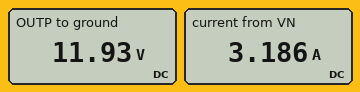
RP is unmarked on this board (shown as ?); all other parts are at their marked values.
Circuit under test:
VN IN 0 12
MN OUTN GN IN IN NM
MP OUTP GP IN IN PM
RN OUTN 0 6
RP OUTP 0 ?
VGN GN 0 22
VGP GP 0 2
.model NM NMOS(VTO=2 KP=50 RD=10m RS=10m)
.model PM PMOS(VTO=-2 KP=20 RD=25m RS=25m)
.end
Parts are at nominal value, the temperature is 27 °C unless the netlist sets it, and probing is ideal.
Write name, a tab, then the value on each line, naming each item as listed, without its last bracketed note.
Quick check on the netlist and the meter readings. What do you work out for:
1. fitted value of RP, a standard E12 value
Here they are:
fitted value of RP, a standard E12 value	10 Ω
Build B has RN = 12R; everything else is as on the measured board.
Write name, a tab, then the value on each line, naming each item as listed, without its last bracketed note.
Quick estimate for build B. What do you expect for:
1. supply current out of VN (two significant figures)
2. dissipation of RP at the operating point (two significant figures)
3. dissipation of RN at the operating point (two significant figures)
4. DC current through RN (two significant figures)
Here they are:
supply current out of VN	2.2 A
dissipation of RP at the operating point	14 W
dissipation of RN at the operating point	12 W
DC current through RN	1.0 A
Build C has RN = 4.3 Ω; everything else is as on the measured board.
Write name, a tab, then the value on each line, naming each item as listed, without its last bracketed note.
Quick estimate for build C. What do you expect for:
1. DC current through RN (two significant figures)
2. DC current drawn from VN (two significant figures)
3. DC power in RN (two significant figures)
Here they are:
DC current through RN	2.8 A
DC current drawn from VN	4.0 A
DC power in RN	33 W
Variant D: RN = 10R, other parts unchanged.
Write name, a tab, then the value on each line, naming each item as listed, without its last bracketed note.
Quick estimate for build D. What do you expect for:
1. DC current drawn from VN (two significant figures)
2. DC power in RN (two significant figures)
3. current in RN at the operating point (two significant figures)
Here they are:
DC current drawn from VN	2.4 A
DC power in RN	14 W
current in RN at the operating point	1.2 A
